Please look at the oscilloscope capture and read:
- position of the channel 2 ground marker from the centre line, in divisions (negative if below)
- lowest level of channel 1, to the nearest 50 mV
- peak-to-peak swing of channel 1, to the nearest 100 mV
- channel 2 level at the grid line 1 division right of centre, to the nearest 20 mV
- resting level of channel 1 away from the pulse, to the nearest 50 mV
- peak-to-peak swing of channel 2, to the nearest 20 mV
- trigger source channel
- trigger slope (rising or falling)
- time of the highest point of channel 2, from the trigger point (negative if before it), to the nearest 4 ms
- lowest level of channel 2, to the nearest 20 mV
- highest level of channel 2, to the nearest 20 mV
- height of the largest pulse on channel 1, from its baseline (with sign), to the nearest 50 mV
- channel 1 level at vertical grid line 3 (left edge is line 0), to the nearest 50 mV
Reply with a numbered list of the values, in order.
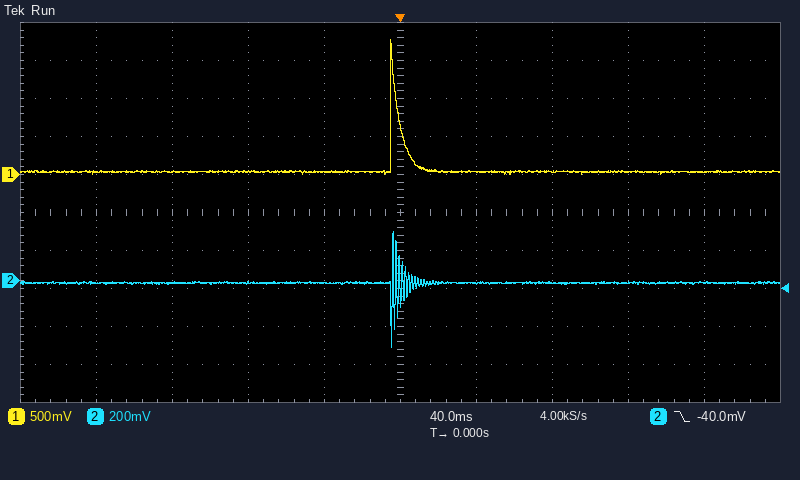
1. -1.8 div
2. 0 mV
3. 1.80 V
4. -20 mV
5. 50 mV
6. 620 mV
7. channel 2
8. falling
9. -4 ms
10. -360 mV
11. 260 mV
12. +1.75 V
13. 50 mV
